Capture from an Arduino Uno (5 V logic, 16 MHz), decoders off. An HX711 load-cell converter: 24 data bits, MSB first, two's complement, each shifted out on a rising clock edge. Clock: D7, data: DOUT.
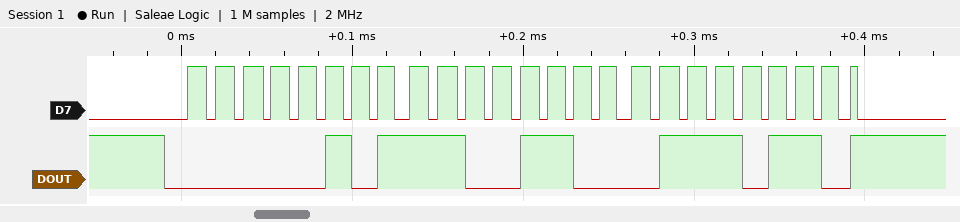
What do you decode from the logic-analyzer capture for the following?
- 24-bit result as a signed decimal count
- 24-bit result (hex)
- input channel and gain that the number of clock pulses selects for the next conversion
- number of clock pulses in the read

380022
0x05CC76
channel A, gain 128
25
